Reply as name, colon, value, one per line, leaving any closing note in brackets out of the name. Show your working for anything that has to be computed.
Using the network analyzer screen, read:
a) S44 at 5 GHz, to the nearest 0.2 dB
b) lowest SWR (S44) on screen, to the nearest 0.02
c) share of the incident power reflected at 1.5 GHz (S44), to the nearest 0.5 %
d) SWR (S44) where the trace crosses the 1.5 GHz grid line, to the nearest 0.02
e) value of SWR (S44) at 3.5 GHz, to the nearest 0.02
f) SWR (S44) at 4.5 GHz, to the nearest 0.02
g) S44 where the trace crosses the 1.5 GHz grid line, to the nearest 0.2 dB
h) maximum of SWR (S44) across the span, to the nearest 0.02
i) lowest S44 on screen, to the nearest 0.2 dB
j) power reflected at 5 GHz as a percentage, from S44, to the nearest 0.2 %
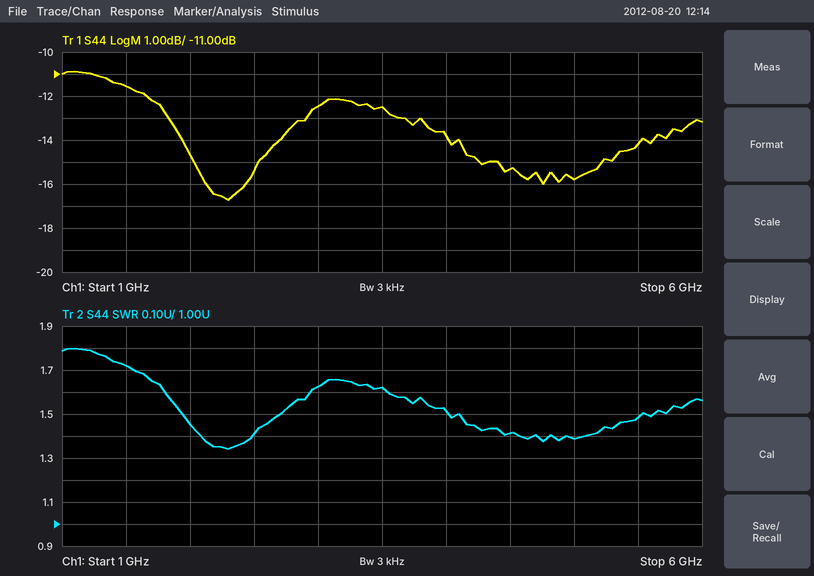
S44 at 5 GHz, to the nearest 0.2 dB: -15.8 dB
lowest SWR (S44) on screen, to the nearest 0.02: 1.34
share of the incident power reflected at 1.5 GHz (S44), to the nearest 0.5 %: 10^(-11.6/10) ≈ 6.92 %, so 7.0 % to the nearest 0.5 %
SWR (S44) where the trace crosses the 1.5 GHz grid line, to the nearest 0.02: 1.72
value of SWR (S44) at 3.5 GHz, to the nearest 0.02: 1.62
SWR (S44) at 4.5 GHz, to the nearest 0.02: 1.42
S44 where the trace crosses the 1.5 GHz grid line, to the nearest 0.2 dB: -11.6 dB
maximum of SWR (S44) across the span, to the nearest 0.02: 1.80
lowest S44 on screen, to the nearest 0.2 dB: -16.8 dB
power reflected at 5 GHz as a percentage, from S44, to the nearest 0.2 %: 10^(-15.8/10) ≈ 2.6 %
